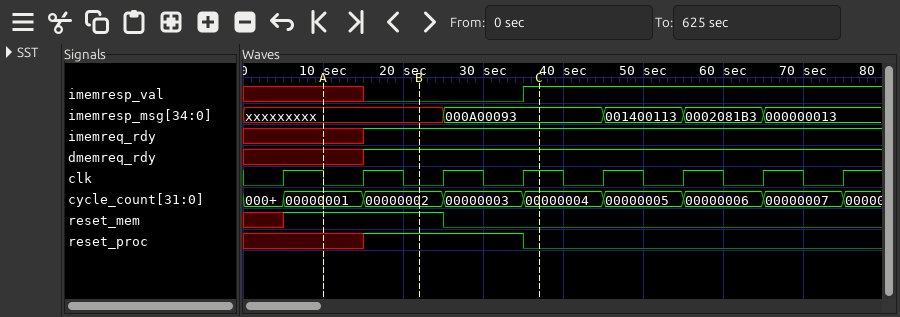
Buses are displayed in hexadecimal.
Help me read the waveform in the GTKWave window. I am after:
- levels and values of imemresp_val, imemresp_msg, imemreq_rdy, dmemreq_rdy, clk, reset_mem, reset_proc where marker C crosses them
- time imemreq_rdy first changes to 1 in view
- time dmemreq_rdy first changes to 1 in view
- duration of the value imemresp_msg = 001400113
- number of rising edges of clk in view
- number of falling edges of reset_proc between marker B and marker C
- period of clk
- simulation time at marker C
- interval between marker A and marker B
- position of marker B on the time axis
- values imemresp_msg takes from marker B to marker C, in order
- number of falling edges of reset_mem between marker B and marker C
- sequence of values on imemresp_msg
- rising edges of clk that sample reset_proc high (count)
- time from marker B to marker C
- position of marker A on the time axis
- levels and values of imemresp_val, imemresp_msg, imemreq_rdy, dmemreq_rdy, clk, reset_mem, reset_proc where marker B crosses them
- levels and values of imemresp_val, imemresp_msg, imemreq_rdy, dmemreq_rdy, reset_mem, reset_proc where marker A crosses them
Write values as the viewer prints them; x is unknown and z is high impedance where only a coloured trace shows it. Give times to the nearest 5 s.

imemresp_val=1, imemresp_msg=000A00093, imemreq_rdy=1, dmemreq_rdy=1, clk=1, reset_mem=0, reset_proc=0
15 s
15 s
10 s
8
1
10 s
35 s
10 s
20 s
xxxxxxxxx, 000A00093
1
xxxxxxxxx, 000A00093, 001400113, 0002081B3, 000000013
2
15 s
10 s
imemresp_val=0, imemresp_msg=xxxxxxxxx, imemreq_rdy=1, dmemreq_rdy=1, clk=0, reset_mem=1, reset_proc=1
imemresp_val=x, imemresp_msg=xxxxxxxxx, imemreq_rdy=x, dmemreq_rdy=x, reset_mem=1, reset_proc=x
